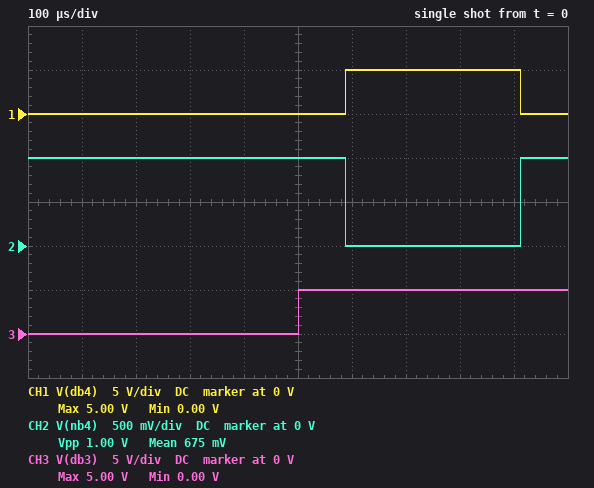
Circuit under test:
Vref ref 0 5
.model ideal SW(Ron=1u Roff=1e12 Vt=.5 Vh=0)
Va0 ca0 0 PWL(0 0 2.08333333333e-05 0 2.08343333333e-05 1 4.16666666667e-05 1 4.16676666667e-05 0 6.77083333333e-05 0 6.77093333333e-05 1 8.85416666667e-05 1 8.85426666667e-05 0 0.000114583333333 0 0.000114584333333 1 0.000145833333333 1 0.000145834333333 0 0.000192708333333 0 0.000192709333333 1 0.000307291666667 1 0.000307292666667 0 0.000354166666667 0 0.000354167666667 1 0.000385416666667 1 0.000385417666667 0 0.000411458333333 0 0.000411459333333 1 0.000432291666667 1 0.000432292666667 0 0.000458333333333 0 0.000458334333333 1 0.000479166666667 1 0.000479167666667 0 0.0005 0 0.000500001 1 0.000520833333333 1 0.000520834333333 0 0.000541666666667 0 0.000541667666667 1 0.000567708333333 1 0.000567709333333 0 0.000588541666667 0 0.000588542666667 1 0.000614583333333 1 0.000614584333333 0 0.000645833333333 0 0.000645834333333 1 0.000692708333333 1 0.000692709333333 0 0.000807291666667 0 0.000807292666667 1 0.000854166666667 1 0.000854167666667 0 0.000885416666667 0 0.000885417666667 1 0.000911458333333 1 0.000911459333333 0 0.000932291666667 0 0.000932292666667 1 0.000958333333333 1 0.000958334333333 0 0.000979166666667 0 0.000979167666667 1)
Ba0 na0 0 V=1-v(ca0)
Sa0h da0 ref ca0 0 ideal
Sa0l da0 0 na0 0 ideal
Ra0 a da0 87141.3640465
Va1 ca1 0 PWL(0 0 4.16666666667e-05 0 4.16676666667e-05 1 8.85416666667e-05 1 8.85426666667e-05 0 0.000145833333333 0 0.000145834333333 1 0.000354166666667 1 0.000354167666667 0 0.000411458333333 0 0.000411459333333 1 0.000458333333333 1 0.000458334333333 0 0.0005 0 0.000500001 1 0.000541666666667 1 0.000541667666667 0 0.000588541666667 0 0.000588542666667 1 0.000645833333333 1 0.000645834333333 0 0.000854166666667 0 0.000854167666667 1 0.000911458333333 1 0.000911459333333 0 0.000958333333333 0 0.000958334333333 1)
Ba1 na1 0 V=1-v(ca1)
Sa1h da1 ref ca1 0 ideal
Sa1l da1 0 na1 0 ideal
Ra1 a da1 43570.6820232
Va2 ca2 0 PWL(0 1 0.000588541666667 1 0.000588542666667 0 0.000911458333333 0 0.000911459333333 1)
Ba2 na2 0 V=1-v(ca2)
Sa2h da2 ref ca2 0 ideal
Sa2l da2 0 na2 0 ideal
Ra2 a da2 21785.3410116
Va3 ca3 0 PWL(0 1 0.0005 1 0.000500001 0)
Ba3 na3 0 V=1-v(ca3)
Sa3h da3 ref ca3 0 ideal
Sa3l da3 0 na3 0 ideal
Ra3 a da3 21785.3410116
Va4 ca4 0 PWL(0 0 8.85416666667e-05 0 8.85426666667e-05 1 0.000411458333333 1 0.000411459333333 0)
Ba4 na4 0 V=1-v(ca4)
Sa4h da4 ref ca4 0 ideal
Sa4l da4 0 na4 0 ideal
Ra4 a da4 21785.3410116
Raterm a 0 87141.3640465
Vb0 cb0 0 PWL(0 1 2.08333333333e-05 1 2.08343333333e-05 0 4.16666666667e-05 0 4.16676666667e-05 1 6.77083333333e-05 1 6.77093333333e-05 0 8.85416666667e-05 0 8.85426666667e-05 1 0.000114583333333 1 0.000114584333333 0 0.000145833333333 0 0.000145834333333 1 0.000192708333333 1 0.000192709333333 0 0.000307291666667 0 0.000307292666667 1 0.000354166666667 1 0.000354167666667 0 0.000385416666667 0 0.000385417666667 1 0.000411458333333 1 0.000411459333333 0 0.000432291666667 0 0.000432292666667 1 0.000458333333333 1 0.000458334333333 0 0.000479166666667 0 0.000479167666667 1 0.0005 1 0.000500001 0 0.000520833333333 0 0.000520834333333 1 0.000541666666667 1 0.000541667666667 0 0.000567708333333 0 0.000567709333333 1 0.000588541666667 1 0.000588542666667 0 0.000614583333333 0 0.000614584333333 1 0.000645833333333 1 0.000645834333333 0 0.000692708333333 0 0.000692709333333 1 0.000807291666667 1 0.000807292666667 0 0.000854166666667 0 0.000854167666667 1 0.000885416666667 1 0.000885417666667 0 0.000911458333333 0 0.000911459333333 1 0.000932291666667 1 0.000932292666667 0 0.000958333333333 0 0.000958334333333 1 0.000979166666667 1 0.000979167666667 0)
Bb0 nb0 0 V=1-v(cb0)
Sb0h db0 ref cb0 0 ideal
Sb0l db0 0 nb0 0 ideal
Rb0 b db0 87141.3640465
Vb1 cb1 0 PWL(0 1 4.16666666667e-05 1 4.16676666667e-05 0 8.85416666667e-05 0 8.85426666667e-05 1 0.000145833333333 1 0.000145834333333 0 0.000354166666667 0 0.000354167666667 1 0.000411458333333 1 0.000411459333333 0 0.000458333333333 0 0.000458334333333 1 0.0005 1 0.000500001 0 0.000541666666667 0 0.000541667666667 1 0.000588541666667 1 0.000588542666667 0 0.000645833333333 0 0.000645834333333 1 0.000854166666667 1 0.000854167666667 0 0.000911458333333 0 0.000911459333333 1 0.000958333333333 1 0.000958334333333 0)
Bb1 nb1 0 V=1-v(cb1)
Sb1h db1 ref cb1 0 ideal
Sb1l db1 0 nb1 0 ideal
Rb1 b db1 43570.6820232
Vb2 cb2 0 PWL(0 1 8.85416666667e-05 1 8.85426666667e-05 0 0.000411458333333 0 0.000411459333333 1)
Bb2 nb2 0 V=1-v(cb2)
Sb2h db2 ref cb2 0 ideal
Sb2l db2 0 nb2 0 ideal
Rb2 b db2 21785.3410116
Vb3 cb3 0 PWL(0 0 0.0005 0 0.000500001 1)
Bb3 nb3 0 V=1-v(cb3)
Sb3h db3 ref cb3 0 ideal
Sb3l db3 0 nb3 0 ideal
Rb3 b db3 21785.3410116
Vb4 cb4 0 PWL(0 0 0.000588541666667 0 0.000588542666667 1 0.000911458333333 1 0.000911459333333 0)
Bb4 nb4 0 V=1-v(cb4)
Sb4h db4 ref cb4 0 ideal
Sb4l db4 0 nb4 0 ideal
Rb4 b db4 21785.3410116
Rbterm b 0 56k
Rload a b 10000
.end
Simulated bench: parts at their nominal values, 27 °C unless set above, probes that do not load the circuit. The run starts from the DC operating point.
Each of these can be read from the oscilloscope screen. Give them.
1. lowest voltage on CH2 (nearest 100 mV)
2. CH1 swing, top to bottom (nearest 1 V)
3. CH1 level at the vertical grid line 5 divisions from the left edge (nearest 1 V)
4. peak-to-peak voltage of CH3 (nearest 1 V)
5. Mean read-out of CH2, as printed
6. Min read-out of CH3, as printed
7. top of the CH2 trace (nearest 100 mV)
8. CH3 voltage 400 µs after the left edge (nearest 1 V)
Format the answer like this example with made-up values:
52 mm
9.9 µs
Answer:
0 V
5 V
0 V
5 V
675 mV
0.00 V
1.0 V
0 V
